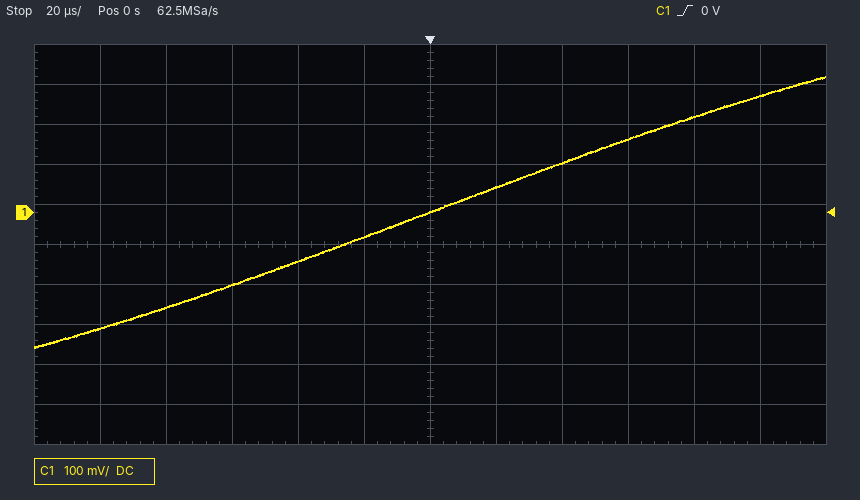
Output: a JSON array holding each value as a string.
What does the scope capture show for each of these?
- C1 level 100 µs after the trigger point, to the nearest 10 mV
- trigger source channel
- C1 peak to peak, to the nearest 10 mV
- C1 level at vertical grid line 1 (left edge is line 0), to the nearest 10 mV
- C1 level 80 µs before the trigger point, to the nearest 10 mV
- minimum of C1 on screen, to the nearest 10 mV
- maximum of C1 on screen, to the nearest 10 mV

["290 mV", "C1", "680 mV", "-290 mV", "-240 mV", "-340 mV", "340 mV"]
